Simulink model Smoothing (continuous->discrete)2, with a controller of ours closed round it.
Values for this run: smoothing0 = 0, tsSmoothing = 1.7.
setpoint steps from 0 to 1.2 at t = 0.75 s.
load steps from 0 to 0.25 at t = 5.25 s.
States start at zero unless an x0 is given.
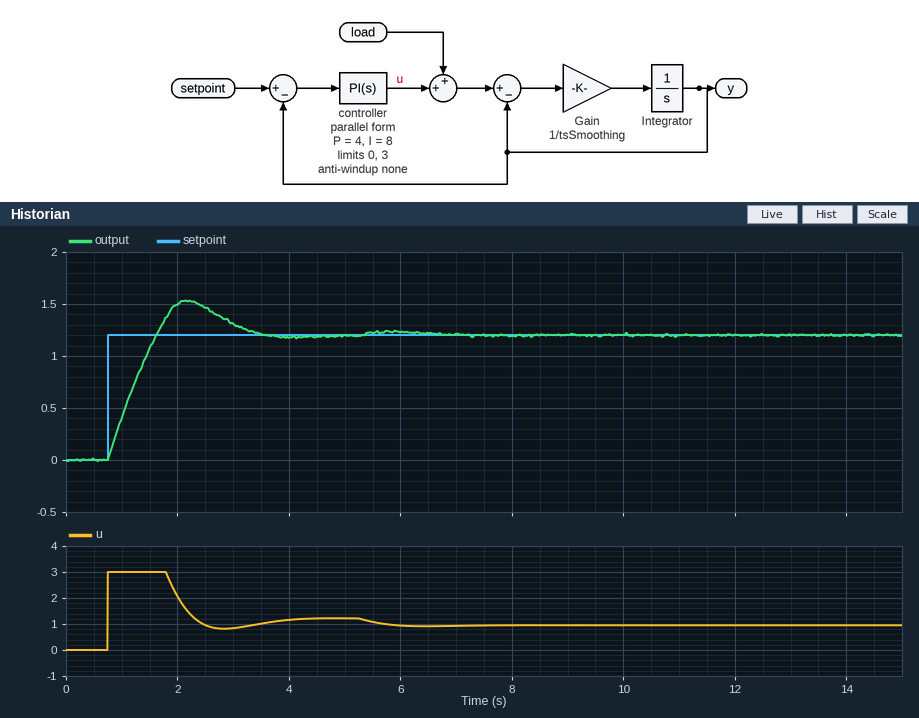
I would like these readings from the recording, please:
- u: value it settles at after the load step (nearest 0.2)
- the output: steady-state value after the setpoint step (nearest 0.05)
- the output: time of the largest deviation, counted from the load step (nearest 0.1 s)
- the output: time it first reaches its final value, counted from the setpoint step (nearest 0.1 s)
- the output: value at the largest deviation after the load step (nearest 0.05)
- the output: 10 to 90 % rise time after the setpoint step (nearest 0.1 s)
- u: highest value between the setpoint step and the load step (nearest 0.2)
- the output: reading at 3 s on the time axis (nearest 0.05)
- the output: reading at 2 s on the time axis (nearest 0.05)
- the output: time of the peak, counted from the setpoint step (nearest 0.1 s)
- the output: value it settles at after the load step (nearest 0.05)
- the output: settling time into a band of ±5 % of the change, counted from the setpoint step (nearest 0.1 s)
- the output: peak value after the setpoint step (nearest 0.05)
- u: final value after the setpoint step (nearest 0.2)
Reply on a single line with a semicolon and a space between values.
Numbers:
1.0; 1.20; 0.5 s; 0.9 s; 1.25; 0.7 s; 3.0; 1.30; 1.50; 1.4 s; 1.20; 2.5 s; 1.55; 1.2
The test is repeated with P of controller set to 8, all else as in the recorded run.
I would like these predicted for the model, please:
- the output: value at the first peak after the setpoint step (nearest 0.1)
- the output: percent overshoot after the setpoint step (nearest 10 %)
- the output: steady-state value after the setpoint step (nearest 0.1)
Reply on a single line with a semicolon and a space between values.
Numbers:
1.4; 20 %; 1.2
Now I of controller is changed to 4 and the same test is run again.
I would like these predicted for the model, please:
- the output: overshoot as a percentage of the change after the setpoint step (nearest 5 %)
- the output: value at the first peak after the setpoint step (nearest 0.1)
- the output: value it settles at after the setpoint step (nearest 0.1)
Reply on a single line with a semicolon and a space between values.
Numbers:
10 %; 1.3; 1.2
